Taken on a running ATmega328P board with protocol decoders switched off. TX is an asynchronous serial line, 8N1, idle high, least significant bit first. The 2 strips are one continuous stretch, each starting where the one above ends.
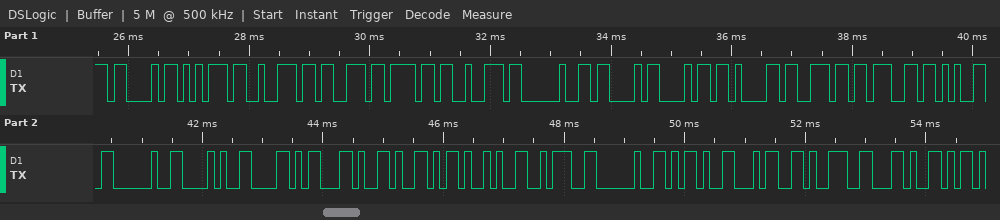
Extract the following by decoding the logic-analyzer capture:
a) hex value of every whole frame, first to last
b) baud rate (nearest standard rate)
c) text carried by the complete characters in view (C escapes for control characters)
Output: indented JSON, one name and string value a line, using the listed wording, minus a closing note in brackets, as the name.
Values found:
{
  "hex value of every whole frame, first to last": "43 75 72 73 6F 72 20 43 68 61 6E 67 65 20 28 58 2C 59 29 3A 20 2D 34 39 2C",
  "baud rate": "9600 baud",
  "text carried by the complete characters in view": "\"Cursor Change (X,Y): -49,\""
}
